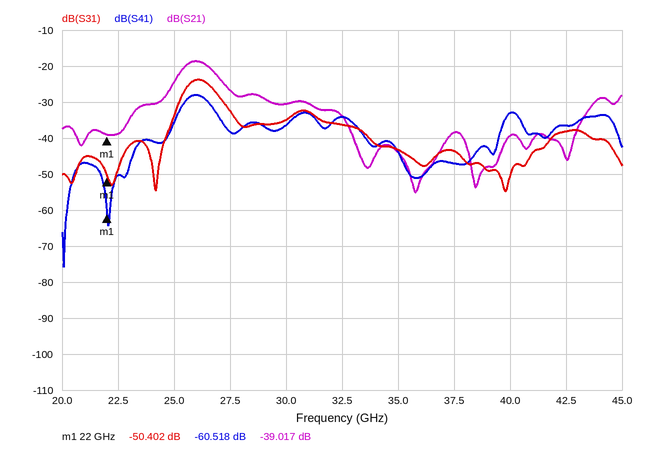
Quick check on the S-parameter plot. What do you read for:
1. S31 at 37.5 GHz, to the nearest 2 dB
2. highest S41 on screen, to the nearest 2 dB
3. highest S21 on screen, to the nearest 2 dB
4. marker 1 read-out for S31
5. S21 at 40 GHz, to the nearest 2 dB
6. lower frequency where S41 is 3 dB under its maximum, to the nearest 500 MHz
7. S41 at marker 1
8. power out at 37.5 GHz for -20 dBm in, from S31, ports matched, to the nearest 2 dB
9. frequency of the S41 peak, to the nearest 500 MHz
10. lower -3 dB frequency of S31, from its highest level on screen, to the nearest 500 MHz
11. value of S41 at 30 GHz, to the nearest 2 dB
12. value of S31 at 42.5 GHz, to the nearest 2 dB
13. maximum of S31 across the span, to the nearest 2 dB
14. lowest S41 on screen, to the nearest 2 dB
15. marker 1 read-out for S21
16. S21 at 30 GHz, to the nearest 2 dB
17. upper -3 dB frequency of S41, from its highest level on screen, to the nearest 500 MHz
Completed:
-44 dB
-28 dB
-18 dB
-50.402 dB
-40 dB
25.5 GHz
-60.518 dB
-64 dBm
26.0 GHz
25.5 GHz
-36 dB
-38 dB
-24 dB
-76 dB
-39.017 dB
-30 dB
26.5 GHz
